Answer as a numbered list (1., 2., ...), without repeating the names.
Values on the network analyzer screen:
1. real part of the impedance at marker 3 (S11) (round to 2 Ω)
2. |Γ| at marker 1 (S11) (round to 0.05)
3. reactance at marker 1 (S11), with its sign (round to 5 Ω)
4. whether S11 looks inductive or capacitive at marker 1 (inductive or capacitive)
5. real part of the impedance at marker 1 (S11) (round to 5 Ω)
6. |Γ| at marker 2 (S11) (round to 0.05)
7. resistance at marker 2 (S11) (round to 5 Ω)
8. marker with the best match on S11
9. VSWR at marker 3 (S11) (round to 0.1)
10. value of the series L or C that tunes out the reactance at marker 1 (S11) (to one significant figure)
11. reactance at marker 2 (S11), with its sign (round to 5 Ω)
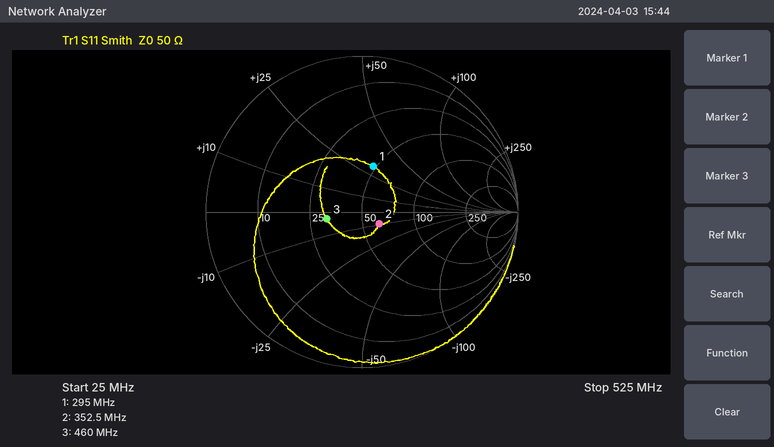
1. 32 Ω
2. 0.30
3. +30 Ω
4. inductive
5. 50 Ω
6. 0.15
7. 60 Ω
8. marker 2
9. 1.6
10. 20 pF
11. -10 Ω
